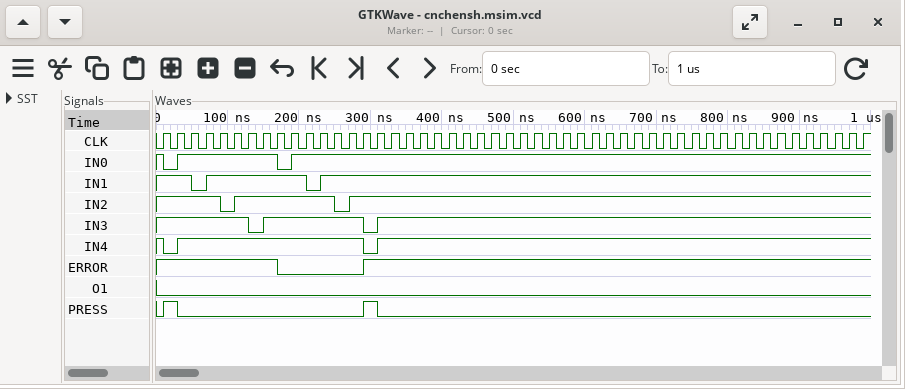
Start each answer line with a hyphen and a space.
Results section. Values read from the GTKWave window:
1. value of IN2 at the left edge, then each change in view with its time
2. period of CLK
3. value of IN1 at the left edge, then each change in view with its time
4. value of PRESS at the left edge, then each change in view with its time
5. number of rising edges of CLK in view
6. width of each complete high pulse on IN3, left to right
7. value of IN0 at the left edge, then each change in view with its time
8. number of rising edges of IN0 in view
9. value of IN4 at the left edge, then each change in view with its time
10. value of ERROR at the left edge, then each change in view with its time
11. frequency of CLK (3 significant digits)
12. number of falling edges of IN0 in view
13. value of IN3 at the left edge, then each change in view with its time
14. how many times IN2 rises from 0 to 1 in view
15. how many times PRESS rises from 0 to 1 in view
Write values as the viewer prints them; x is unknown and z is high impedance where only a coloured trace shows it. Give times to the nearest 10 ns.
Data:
- 1, 0 at 90 ns, 1 at 110 ns, 0 at 250 ns, 1 at 270 ns
- 20 ns
- 1, 0 at 50 ns, 1 at 70 ns, 0 at 210 ns, 1 at 230 ns
- 0, 1 at 10 ns, 0 at 30 ns, 1 at 290 ns, 0 at 310 ns
- 50
- 140 ns
- 1, 0 at 10 ns, 1 at 30 ns, 0 at 170 ns, 1 at 190 ns
- 2
- 1, 0 at 10 ns, 1 at 30 ns, 0 at 290 ns, 1 at 310 ns
- 1, 0 at 170 ns, 1 at 290 ns
- 50.0 MHz
- 2
- 1, 0 at 130 ns, 1 at 150 ns, 0 at 290 ns, 1 at 310 ns
- 2
- 2
